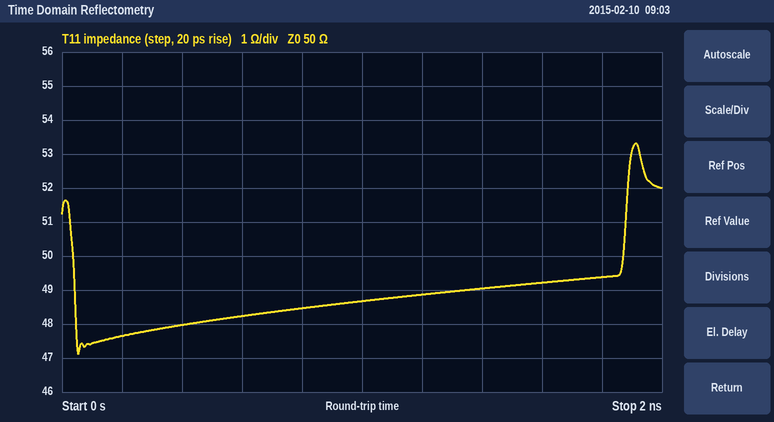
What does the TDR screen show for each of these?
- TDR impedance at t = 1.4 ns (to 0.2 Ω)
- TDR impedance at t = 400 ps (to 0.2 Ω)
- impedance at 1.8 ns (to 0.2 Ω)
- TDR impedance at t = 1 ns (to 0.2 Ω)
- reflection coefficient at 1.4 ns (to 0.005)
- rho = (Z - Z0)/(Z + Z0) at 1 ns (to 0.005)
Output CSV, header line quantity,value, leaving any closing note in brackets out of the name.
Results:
quantity,value
TDR impedance at t = 1.4 ns,49.0 Ω
TDR impedance at t = 400 ps,48.0 Ω
impedance at 1.8 ns,49.4 Ω
TDR impedance at t = 1 ns,48.6 Ω
reflection coefficient at 1.4 ns,-0.010
rho = (Z - Z0)/(Z + Z0) at 1 ns,-0.015
